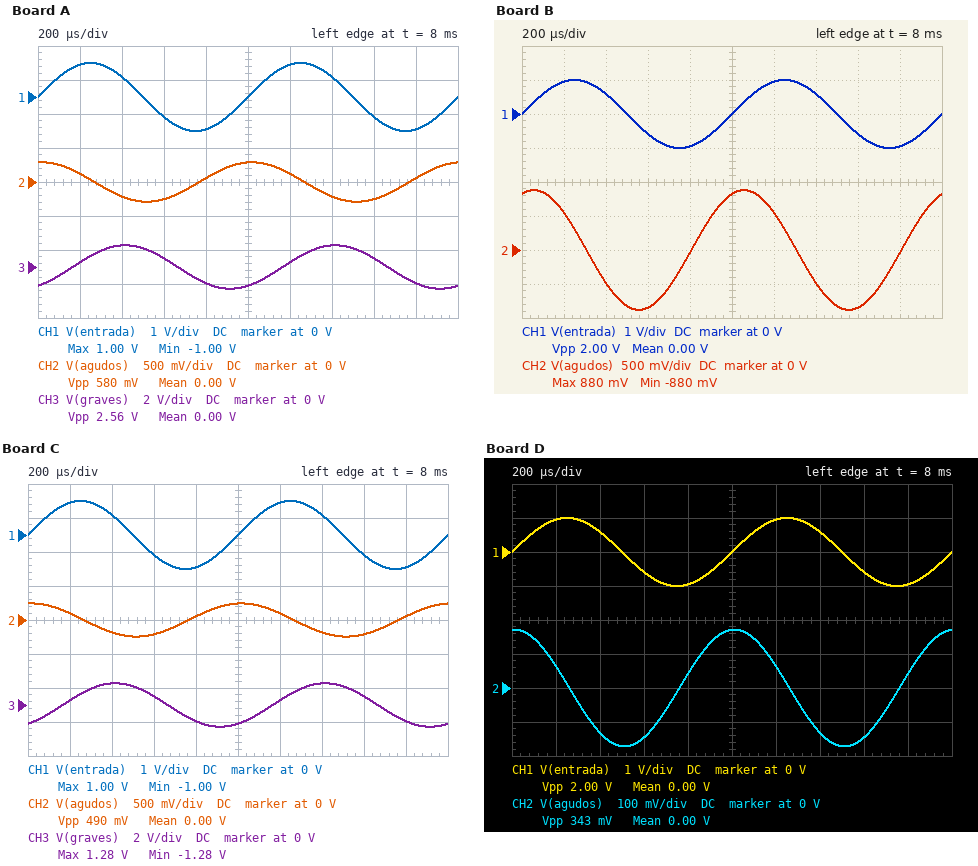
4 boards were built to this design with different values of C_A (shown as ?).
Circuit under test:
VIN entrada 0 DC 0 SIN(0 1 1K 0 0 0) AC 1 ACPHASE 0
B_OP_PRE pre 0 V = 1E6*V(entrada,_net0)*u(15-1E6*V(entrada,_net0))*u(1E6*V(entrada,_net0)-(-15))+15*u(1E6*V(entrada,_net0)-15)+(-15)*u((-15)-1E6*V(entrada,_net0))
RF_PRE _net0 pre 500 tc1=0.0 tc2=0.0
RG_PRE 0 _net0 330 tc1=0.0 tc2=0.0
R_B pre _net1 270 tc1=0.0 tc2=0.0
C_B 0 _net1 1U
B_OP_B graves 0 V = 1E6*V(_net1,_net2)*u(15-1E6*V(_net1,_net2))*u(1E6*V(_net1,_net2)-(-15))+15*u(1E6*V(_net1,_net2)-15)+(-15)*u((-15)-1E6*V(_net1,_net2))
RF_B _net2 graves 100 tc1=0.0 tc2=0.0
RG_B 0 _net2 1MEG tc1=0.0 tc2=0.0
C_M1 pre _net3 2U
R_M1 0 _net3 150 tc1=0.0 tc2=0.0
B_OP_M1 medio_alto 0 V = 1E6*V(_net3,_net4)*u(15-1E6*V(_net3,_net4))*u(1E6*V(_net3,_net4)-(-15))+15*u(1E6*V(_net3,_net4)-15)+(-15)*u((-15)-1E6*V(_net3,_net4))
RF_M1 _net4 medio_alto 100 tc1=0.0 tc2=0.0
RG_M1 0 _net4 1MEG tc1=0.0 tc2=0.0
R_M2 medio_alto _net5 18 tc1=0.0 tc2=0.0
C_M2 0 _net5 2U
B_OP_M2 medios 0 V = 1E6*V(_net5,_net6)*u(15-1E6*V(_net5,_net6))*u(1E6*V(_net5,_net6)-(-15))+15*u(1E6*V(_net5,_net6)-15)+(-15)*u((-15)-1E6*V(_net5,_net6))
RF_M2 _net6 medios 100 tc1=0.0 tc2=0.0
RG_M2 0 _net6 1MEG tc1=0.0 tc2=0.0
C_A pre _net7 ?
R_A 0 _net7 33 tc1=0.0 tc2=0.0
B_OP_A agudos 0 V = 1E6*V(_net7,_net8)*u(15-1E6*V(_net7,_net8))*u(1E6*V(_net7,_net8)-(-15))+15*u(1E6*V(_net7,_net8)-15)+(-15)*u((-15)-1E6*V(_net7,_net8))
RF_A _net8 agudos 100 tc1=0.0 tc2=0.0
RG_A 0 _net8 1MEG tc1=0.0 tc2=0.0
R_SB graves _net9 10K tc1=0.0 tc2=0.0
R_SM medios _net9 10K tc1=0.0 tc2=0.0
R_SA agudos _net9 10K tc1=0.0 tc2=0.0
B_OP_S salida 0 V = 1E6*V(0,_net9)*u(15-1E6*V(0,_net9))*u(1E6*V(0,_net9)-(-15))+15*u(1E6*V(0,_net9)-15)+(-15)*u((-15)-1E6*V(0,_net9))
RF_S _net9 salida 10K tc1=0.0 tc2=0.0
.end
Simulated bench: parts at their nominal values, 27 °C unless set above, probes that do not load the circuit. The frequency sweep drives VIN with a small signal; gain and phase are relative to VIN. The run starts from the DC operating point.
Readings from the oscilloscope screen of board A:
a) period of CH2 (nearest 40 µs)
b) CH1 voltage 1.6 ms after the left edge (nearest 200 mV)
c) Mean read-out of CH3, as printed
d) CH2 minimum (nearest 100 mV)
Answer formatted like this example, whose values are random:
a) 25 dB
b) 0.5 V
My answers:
a) 1.00 ms
b) -600 mV
c) 0.00 V
d) -300 mV
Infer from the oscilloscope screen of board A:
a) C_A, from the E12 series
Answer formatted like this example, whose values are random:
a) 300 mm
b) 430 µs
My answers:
a) 560 nF
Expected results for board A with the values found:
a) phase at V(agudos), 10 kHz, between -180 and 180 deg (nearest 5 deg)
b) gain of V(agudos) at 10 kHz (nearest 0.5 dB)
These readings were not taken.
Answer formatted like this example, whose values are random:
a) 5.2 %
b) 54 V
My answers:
a) 40 deg
b) 5.5 dB
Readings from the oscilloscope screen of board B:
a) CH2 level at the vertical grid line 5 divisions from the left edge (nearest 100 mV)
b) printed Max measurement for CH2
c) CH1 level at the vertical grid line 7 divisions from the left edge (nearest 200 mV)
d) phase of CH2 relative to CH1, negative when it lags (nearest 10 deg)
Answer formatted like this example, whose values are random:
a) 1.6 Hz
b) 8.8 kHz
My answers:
a) 800 mV
b) 880 mV
c) 600 mV
d) 70 deg
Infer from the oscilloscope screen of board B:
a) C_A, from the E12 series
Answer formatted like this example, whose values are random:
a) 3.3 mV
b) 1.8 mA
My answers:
a) 1.8 µF
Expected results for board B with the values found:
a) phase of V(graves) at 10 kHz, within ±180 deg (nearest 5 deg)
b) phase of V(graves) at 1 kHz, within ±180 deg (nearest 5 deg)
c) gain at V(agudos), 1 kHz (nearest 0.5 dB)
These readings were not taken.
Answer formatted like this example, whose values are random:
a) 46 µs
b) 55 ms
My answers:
a) -85 deg
b) -60 deg
c) -1.0 dB
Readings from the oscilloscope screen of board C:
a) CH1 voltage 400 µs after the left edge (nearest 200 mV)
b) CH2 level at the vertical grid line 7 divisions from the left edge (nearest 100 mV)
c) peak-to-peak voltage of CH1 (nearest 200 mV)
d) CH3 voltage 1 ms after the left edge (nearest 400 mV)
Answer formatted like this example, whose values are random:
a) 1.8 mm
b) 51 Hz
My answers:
a) 600 mV
b) -200 mV
c) 2.0 V
d) -1.2 V
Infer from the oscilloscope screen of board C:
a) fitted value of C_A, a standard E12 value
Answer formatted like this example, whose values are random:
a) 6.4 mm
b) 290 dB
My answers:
a) 470 nF
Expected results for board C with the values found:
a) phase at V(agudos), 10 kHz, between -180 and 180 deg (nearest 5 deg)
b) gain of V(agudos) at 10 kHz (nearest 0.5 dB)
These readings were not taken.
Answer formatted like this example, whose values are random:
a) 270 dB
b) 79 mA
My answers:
a) 45 deg
b) 5.0 dB
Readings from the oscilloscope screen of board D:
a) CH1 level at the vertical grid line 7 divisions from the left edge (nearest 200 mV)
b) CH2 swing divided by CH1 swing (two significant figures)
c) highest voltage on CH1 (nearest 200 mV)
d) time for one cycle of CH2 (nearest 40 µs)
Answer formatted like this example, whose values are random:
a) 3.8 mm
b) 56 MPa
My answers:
a) 600 mV
b) 0.17
c) 1.0 V
d) 1.00 ms
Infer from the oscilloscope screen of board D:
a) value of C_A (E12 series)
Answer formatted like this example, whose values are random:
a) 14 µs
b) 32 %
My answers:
a) 330 nF
